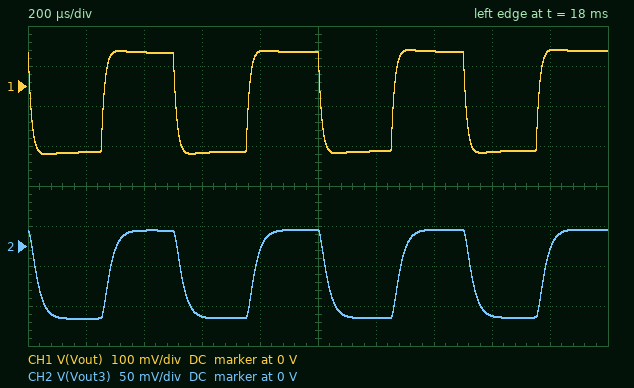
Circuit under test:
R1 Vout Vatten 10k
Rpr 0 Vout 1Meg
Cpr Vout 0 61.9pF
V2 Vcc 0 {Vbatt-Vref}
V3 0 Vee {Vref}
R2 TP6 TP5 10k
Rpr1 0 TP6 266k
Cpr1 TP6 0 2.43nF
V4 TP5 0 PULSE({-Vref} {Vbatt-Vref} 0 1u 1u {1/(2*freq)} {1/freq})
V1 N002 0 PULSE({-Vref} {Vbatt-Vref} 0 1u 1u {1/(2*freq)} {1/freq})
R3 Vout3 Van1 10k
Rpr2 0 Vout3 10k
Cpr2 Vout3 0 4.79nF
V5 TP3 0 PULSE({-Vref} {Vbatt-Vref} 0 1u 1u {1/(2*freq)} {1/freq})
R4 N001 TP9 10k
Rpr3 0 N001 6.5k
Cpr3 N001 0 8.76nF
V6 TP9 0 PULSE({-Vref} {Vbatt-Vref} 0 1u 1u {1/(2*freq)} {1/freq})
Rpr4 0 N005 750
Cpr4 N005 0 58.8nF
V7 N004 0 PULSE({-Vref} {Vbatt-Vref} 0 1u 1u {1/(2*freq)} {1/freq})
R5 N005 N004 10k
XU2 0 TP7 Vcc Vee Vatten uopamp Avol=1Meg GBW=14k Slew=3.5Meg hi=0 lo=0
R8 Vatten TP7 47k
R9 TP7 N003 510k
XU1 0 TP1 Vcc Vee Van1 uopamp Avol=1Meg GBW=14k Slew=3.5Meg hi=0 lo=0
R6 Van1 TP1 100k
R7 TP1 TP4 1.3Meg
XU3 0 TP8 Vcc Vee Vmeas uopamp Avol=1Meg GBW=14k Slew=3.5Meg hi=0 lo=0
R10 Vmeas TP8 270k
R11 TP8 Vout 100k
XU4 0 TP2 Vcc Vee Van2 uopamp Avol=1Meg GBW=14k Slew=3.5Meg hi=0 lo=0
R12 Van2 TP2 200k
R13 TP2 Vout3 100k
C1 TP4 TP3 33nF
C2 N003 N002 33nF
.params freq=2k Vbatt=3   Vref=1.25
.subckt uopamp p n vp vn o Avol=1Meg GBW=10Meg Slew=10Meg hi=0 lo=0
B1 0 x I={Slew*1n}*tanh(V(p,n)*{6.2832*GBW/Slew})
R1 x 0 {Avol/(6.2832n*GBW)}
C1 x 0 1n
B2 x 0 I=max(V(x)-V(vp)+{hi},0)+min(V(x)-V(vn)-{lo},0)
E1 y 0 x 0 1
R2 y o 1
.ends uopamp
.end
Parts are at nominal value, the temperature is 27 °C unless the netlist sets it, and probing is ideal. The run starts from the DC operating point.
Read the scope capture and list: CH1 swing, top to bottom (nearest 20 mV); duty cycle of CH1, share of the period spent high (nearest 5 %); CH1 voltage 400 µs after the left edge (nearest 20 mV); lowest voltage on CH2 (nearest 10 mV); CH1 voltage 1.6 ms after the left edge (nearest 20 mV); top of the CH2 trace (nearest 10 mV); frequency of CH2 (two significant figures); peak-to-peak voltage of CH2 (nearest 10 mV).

260 mV
50 %
80 mV
-90 mV
-160 mV
20 mV
2.0 kHz
110 mV
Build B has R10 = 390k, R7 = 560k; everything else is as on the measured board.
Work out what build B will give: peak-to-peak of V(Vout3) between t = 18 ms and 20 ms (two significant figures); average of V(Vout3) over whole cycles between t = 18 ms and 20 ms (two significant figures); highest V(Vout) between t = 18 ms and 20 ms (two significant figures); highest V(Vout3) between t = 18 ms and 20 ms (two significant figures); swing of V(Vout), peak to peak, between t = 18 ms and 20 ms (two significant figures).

260 mV
-46 mV
93 mV
85 mV
270 mV
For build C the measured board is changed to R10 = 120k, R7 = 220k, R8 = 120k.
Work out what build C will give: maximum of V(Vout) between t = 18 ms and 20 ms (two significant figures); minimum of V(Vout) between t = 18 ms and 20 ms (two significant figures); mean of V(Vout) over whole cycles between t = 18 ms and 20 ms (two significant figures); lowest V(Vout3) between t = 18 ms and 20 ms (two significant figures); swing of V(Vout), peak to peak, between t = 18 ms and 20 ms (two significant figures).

220 mV
-430 mV
-100 mV
-350 mV
650 mV
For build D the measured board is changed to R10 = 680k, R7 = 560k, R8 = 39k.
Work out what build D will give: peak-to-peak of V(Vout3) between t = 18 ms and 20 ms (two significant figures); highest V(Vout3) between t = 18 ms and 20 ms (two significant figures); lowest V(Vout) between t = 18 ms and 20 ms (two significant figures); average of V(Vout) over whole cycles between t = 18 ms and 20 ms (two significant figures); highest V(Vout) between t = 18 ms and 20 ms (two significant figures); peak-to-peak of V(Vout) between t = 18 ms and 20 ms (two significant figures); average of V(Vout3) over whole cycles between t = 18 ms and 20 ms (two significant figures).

260 mV
85 mV
-150 mV
-33 mV
80 mV
230 mV
-46 mV
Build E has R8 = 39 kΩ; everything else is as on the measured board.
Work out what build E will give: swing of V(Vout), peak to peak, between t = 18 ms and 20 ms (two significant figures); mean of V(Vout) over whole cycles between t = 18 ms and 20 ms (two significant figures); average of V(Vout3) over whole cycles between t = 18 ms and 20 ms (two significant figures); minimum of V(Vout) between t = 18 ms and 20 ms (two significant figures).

220 mV
-33 mV
-35 mV
-140 mV
